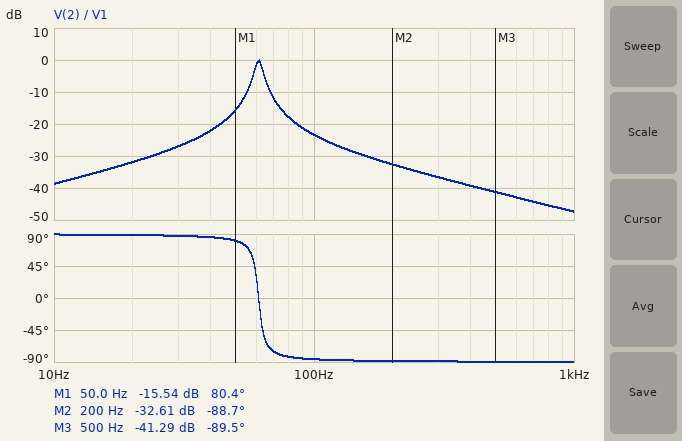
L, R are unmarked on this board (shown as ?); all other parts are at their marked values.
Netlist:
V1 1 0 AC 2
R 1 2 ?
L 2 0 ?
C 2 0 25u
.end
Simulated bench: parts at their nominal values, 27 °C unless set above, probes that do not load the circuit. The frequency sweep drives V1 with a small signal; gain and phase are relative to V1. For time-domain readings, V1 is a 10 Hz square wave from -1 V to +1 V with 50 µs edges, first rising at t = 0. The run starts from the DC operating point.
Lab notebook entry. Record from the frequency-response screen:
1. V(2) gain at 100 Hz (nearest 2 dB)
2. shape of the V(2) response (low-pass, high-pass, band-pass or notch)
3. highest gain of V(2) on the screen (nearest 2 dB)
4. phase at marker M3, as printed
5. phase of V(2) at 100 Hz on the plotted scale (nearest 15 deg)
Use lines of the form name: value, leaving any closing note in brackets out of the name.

V(2) gain at 100 Hz: -24 dB
shape of the V(2) response: band-pass
highest gain of V(2) on the screen: 0 dB
phase at marker M3, as printed: -89.5 deg
phase of V(2) at 100 Hz on the plotted scale: -90 deg
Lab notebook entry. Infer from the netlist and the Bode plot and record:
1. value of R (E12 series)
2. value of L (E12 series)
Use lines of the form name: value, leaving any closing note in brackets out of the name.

value of R: 1.5 kΩ
value of L: 270 mH
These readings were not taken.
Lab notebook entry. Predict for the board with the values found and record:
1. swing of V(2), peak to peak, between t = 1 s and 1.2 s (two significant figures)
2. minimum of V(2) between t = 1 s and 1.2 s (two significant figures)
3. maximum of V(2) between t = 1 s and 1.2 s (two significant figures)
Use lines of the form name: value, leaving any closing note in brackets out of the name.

swing of V(2), peak to peak, between t = 1 s and 1.2 s: 180 mV
minimum of V(2) between t = 1 s and 1.2 s: -88 mV
maximum of V(2) between t = 1 s and 1.2 s: 88 mV
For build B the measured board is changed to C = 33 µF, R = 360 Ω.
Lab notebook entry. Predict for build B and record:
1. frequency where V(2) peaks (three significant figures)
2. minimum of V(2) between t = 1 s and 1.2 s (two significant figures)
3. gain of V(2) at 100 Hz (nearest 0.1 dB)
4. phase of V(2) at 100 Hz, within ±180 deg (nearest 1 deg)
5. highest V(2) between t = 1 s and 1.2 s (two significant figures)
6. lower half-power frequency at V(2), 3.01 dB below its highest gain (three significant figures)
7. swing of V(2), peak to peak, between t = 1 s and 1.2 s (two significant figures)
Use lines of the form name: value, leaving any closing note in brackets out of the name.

frequency where V(2) peaks: 53.3 Hz
minimum of V(2) between t = 1 s and 1.2 s: -460 mV
gain of V(2) at 100 Hz: -14.7 dB
phase of V(2) at 100 Hz, within ±180 deg: -79 deg
highest V(2) between t = 1 s and 1.2 s: 460 mV
lower half-power frequency at V(2), 3.01 dB below its highest gain: 47.0 Hz
swing of V(2), peak to peak, between t = 1 s and 1.2 s: 910 mV
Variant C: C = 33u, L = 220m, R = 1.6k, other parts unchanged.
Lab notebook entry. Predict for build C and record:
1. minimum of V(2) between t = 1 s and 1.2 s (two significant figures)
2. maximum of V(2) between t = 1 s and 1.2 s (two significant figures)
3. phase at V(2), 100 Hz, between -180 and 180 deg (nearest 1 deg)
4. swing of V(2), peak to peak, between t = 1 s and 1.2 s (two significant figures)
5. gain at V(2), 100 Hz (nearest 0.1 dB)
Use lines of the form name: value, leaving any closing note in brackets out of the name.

minimum of V(2) between t = 1 s and 1.2 s: -61 mV
maximum of V(2) between t = 1 s and 1.2 s: 61 mV
phase at V(2), 100 Hz, between -180 and 180 deg: -87 deg
swing of V(2), peak to peak, between t = 1 s and 1.2 s: 120 mV
gain at V(2), 100 Hz: -26.7 dB
